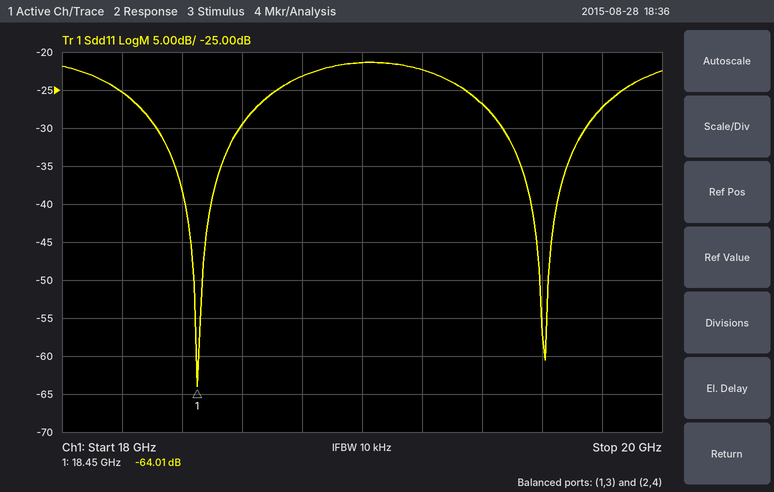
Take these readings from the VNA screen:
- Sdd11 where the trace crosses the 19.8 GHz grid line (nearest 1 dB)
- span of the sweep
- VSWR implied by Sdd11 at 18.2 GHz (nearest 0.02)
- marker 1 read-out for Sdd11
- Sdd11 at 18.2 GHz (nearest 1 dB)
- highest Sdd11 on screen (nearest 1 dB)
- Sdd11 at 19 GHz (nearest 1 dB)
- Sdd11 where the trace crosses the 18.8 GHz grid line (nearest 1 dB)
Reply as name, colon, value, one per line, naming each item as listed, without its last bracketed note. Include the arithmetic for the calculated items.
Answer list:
Sdd11 where the trace crosses the 19.8 GHz grid line: -27 dB
span of the sweep: 2 GHz
VSWR implied by Sdd11 at 18.2 GHz: |Γ| = 10^(-25/20) = 0.0562; VSWR = (1 + 0.0562)/(1 − 0.0562) ≈ 1.12
marker 1 read-out for Sdd11: -64.01 dB
Sdd11 at 18.2 GHz: -25 dB
highest Sdd11 on screen: -21 dB
Sdd11 at 19 GHz: -21 dB
Sdd11 where the trace crosses the 18.8 GHz grid line: -23 dB
